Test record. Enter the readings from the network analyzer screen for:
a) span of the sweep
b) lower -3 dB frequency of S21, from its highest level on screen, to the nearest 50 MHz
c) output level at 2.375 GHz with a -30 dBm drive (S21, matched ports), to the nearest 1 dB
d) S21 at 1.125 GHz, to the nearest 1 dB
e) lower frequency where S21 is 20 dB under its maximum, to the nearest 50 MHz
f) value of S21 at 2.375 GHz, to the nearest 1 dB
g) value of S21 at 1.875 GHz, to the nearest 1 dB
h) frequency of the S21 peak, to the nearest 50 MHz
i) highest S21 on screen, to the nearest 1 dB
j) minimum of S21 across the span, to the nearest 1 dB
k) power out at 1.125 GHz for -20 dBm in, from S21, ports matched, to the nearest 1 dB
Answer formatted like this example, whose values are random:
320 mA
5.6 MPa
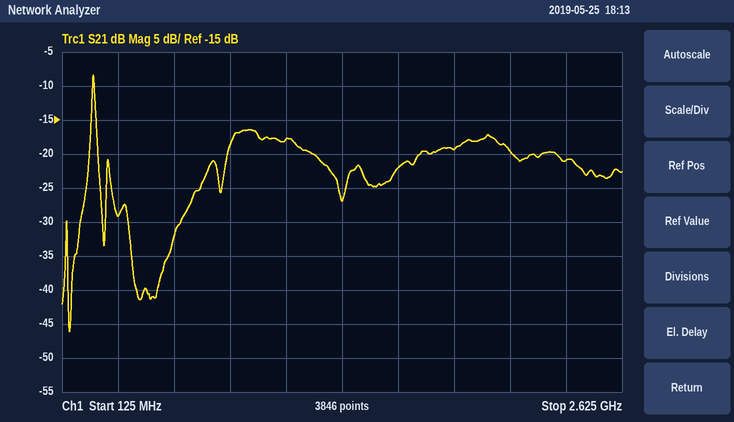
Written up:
2.5 GHz
250 MHz
-51 dBm
-18 dB
200 MHz
-21 dB
-19 dB
250 MHz
-8 dB
-46 dB
-38 dBm
